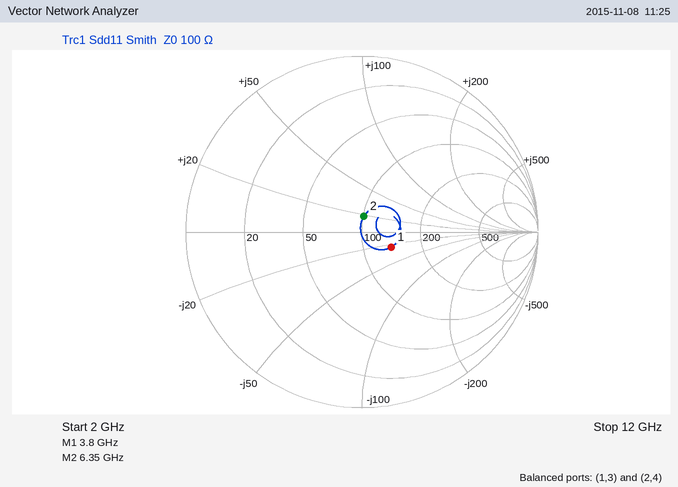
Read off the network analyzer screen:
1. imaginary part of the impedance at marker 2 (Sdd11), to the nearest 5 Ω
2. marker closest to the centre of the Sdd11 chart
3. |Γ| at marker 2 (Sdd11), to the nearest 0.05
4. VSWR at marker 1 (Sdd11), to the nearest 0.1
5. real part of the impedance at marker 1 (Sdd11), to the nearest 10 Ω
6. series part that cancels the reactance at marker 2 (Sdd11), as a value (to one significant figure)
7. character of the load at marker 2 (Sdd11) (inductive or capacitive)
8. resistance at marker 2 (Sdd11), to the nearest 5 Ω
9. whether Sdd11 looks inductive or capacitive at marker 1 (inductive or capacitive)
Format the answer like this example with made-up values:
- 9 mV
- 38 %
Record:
- +20 Ω
- marker 2
- 0.10
- 1.5
- 140 Ω
- 1 pF
- inductive
- 100 Ω
- capacitive
